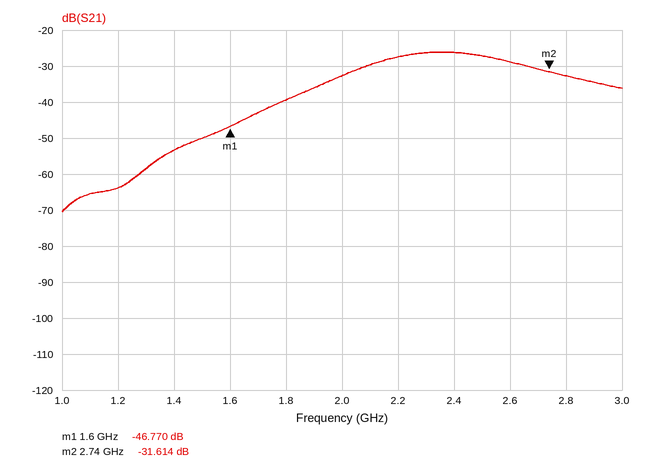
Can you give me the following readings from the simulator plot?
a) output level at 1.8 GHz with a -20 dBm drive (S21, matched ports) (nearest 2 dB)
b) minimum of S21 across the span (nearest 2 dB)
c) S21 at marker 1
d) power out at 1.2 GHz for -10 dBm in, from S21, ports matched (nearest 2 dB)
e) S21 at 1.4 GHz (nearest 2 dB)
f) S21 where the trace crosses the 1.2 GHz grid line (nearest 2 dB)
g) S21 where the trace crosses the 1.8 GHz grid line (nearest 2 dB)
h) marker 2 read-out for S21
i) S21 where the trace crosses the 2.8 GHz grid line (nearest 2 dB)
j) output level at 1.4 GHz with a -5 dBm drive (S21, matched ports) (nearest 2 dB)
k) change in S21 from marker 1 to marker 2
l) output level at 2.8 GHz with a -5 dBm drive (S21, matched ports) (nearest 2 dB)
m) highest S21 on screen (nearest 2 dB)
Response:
-60 dBm
-70 dB
-46.770 dB
-74 dBm
-54 dB
-64 dB
-40 dB
-31.614 dB
-32 dB
-58 dBm
15.156 dB
-38 dBm
-26 dB
